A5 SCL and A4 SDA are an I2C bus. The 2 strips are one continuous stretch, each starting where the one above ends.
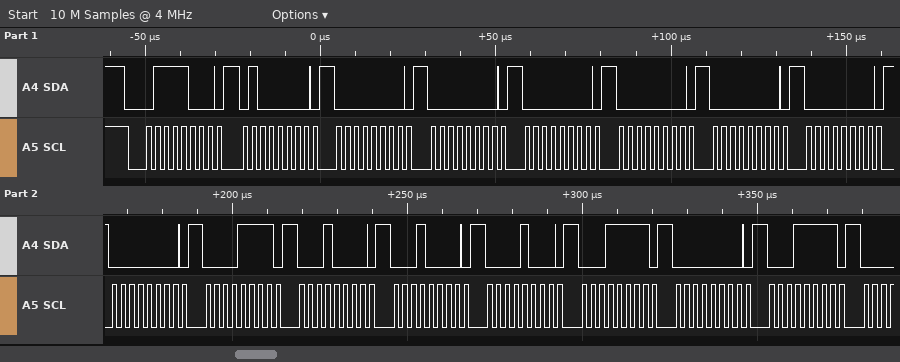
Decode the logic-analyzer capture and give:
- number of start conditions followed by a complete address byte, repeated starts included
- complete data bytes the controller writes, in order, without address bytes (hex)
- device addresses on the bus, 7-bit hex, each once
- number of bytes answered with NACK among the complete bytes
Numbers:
1
40 00 00 00 00 00 00 00 0F 10 10 08 1F 00 1F
0x3C
0
